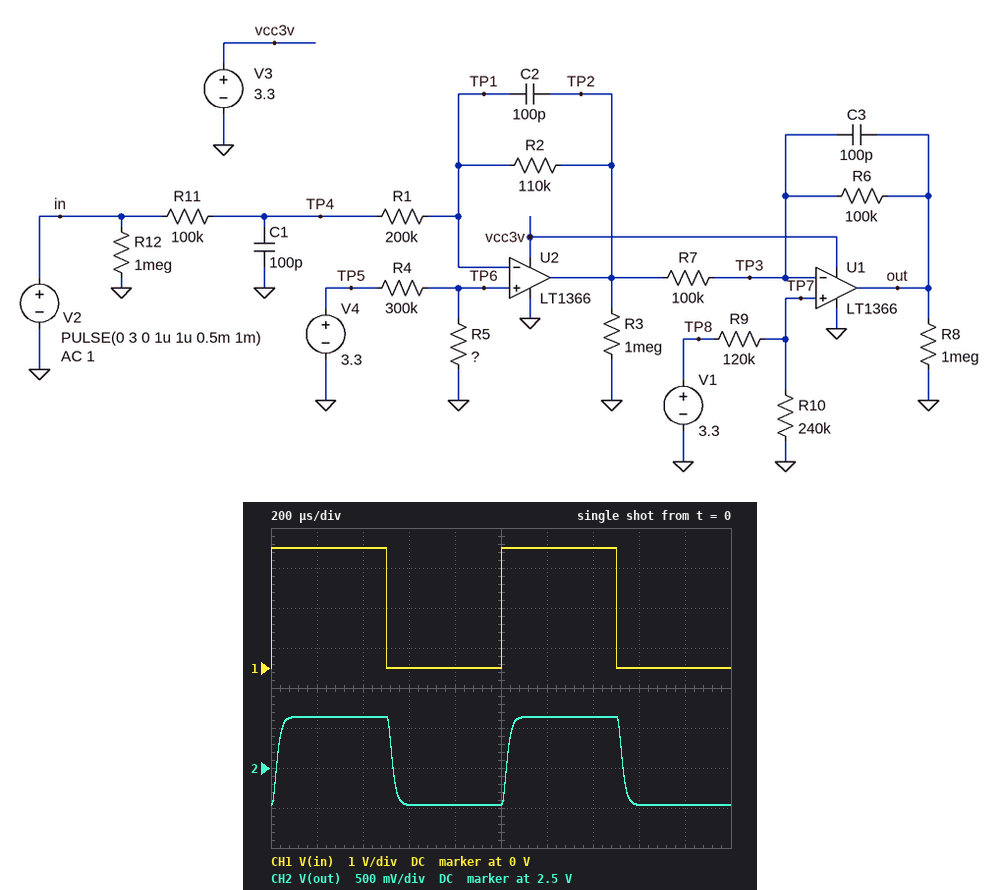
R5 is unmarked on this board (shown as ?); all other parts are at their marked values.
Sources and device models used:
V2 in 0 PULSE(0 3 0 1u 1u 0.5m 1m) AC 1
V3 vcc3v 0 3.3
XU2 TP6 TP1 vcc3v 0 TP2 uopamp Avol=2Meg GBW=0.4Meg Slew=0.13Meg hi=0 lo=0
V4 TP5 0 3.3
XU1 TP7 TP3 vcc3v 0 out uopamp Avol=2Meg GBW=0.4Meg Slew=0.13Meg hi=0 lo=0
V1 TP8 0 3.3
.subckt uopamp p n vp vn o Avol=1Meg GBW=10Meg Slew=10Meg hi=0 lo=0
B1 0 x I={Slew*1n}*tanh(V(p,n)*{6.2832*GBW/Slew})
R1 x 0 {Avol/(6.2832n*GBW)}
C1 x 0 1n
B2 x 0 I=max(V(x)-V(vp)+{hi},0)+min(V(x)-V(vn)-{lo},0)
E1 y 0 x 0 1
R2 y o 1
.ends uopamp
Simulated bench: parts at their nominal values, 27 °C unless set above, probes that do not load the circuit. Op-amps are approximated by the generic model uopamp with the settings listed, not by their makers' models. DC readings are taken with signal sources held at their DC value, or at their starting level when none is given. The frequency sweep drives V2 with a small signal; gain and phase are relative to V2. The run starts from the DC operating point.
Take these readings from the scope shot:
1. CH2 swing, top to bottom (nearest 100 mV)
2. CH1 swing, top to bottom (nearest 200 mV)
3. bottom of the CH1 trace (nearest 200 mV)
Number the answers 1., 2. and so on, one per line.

1. 1.1 V
2. 3.0 V
3. 0 V
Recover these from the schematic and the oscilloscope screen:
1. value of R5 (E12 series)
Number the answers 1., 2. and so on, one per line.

1. 330 kΩ
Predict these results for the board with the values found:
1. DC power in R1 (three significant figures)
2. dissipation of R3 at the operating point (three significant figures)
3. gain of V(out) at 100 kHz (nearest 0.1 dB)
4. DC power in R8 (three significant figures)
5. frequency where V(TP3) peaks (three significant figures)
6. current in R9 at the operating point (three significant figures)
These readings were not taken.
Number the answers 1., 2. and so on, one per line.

1. 6.64 µW
2. 5.58 µW
3. -55.4 dB
4. 4.15 µW
5. 12.0 kHz
6. 9.17 µA
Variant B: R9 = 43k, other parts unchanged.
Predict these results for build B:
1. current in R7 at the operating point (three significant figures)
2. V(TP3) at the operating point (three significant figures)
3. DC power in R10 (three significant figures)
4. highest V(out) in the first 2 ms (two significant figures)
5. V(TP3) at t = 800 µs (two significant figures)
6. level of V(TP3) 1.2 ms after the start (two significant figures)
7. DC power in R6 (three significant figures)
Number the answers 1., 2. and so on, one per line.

1. 4.36 µA
2. 2.80 V
3. 32.6 µW
4. 3.3 V
5. 2.8 V
6. 2.3 V
7. 1.90 µW
